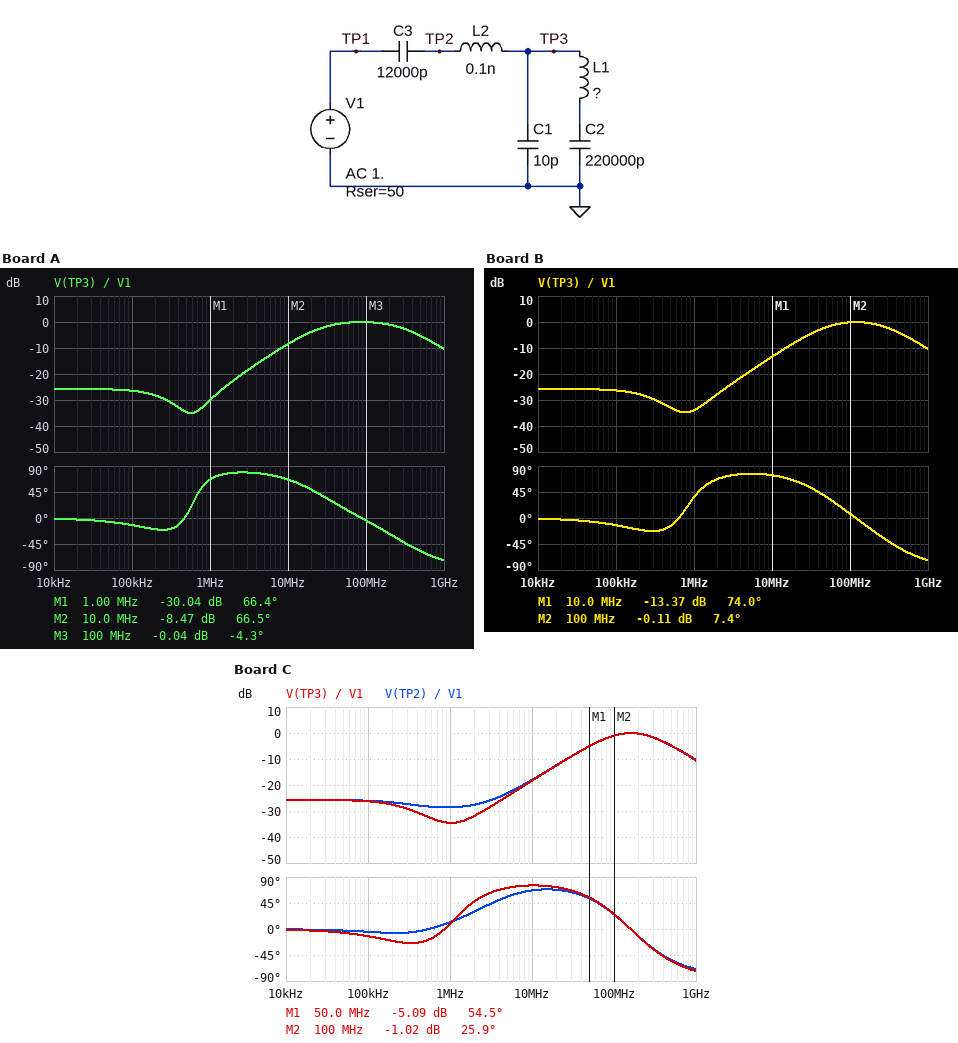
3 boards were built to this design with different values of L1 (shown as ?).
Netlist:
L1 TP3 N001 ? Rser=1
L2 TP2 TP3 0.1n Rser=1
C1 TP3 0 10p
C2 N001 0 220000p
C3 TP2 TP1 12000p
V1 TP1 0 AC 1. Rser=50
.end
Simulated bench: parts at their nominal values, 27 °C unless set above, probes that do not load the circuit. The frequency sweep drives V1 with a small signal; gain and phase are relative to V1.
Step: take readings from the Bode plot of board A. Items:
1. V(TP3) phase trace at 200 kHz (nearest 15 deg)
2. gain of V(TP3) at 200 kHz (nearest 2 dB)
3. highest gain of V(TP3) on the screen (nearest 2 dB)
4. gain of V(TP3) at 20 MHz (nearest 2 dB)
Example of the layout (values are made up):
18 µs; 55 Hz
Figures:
-15 deg; -28 dB; 0 dB; -4 dB
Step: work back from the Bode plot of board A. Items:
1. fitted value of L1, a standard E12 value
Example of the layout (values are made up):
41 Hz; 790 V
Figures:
330 nH
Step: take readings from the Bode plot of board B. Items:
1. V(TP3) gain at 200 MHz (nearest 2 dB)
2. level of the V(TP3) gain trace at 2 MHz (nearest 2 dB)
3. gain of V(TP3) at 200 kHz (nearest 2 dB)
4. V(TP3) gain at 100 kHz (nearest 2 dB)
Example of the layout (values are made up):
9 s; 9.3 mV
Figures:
0 dB; -28 dB; -28 dB; -26 dB
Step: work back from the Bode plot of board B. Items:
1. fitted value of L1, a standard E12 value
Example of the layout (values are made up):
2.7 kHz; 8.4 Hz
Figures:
180 nH
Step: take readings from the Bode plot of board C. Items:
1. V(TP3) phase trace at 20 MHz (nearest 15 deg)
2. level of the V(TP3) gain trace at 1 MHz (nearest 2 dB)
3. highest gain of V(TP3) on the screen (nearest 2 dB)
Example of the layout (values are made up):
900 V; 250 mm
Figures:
75 deg; -34 dB; 0 dB
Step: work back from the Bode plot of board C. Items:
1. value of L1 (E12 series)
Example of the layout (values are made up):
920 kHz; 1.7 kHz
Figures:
100 nH
